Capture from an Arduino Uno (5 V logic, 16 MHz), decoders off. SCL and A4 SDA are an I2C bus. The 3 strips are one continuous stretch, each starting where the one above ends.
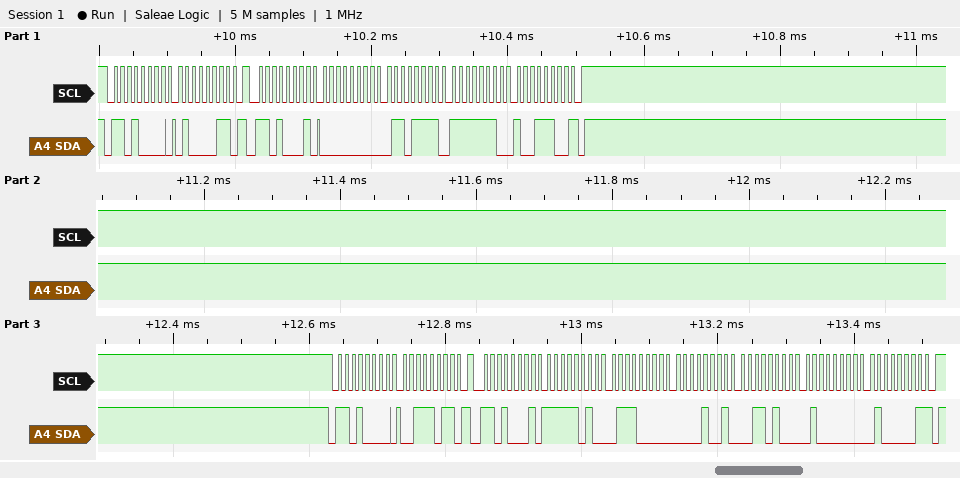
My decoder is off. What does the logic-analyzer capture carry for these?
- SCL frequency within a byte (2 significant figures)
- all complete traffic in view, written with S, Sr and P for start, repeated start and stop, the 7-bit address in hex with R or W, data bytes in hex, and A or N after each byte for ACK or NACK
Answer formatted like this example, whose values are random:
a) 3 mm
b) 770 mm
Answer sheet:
a) 100 kHz
b) S 68W A 43 A Sr 68R A 00 A 6F A FE A 9C N P S 68W A 3B A Sr 68R A FA A 70 A 09 A 34 A 40 A 41 N P
